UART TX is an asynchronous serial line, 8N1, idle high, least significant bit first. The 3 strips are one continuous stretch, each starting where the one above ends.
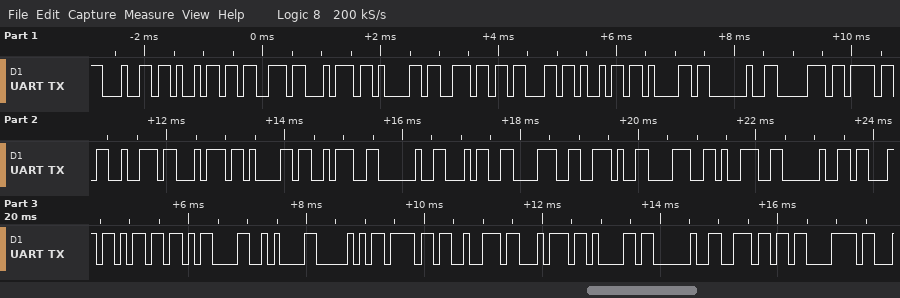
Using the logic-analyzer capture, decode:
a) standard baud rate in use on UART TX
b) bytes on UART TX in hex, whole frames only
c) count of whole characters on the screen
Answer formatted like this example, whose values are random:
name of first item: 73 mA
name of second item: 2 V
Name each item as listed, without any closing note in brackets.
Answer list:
standard baud rate in use on UART TX: 9600 baud
bytes on UART TX in hex, whole frames only: 64 69 73 74 61 6E 63 69 61 20 70 6F 72 74 61 3A 20 34 38 2E 38 39 20 63 6D 0D 0A 50 6F 72 74 61 20 6E C3
count of whole characters on the screen: 35
